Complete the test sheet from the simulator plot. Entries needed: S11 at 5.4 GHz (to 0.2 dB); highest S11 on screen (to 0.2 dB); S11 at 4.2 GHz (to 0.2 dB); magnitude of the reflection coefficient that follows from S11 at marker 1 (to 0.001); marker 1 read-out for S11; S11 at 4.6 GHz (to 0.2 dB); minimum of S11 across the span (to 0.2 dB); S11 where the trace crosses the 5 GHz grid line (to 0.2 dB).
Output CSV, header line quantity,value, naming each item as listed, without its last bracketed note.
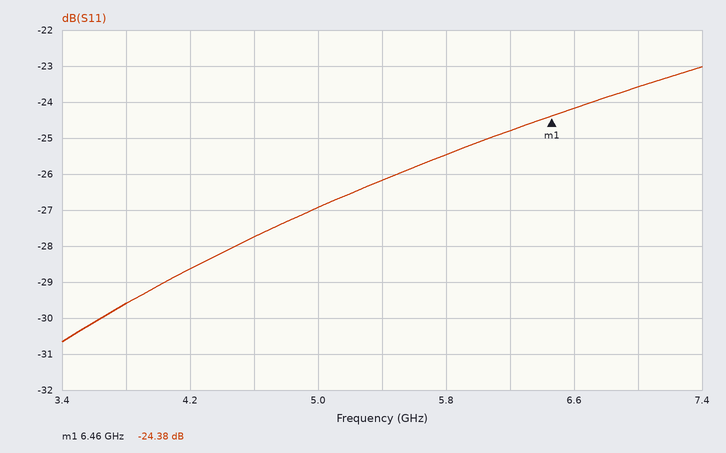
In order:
quantity,value
S11 at 5.4 GHz,-26.2 dB
highest S11 on screen,-23.0 dB
S11 at 4.2 GHz,-28.6 dB
magnitude of the reflection coefficient that follows from S11 at marker 1,0.060
marker 1 read-out for S11,-24.38 dB
S11 at 4.6 GHz,-27.8 dB
minimum of S11 across the span,-30.6 dB
S11 where the trace crosses the 5 GHz grid line,-27.0 dB
